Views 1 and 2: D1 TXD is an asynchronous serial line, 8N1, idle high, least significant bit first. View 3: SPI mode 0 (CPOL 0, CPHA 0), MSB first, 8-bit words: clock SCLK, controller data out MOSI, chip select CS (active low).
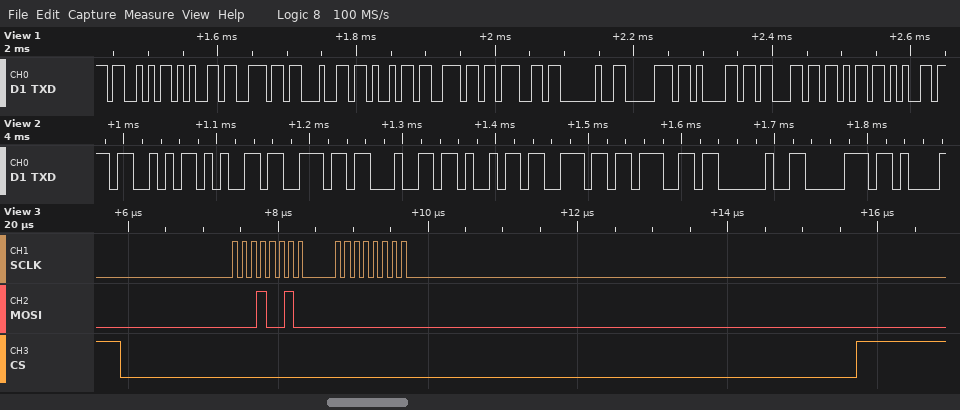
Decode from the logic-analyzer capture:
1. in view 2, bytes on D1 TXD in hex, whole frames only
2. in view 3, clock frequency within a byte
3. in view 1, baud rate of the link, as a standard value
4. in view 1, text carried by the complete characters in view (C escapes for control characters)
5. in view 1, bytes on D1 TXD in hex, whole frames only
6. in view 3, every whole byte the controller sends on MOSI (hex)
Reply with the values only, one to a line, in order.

53 65 6E 64 69 6E 67 20 70
8 MHz
115200 baud
"Sending packe"
53 65 6E 64 69 6E 67 20 70 61 63 6B 65
0x12 0x00
